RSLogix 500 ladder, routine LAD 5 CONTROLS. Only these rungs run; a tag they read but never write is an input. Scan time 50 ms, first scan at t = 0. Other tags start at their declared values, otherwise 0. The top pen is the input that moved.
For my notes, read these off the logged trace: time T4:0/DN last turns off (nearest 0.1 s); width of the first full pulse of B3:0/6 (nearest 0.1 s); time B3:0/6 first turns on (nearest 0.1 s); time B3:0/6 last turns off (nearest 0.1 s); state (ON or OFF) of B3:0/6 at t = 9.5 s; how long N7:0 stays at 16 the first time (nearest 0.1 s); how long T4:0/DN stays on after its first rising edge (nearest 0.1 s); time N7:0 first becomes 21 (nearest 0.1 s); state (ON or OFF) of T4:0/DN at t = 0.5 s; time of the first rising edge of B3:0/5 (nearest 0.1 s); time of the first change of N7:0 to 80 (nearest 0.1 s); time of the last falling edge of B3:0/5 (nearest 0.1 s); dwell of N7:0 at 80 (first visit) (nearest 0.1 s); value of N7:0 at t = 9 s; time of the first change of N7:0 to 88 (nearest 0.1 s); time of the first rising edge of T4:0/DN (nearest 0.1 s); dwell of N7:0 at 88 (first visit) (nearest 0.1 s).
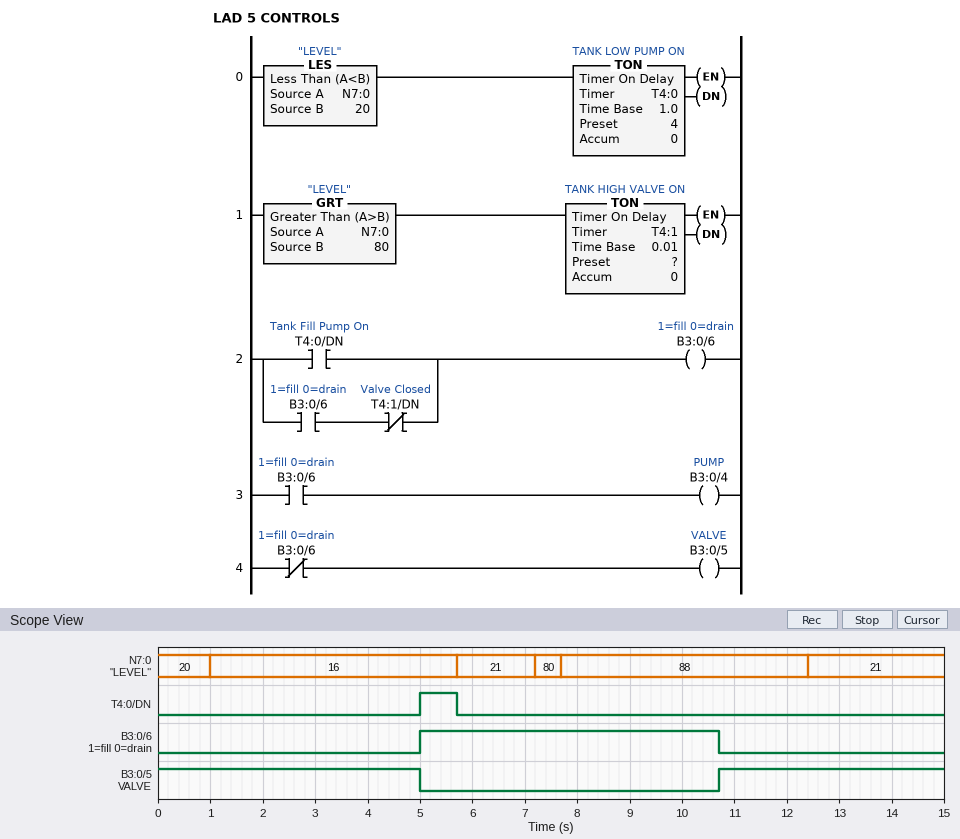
5.7 s
5.7 s
5.0 s
10.7 s
ON
4.7 s
0.7 s
5.7 s
OFF
10.7 s
7.2 s
5.0 s
0.5 s
88
7.7 s
5.0 s
4.7 s
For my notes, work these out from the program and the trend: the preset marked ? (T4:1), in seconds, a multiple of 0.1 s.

3.0 s
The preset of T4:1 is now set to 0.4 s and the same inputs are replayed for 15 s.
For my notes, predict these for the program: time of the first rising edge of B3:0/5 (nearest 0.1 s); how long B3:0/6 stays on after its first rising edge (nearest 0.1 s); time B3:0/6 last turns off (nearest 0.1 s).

8.1 s
3.1 s
8.1 s
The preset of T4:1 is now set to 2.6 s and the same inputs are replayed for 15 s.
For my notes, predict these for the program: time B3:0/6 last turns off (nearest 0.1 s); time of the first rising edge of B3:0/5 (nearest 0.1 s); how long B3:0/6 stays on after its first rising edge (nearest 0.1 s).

10.3 s
10.3 s
5.3 s
